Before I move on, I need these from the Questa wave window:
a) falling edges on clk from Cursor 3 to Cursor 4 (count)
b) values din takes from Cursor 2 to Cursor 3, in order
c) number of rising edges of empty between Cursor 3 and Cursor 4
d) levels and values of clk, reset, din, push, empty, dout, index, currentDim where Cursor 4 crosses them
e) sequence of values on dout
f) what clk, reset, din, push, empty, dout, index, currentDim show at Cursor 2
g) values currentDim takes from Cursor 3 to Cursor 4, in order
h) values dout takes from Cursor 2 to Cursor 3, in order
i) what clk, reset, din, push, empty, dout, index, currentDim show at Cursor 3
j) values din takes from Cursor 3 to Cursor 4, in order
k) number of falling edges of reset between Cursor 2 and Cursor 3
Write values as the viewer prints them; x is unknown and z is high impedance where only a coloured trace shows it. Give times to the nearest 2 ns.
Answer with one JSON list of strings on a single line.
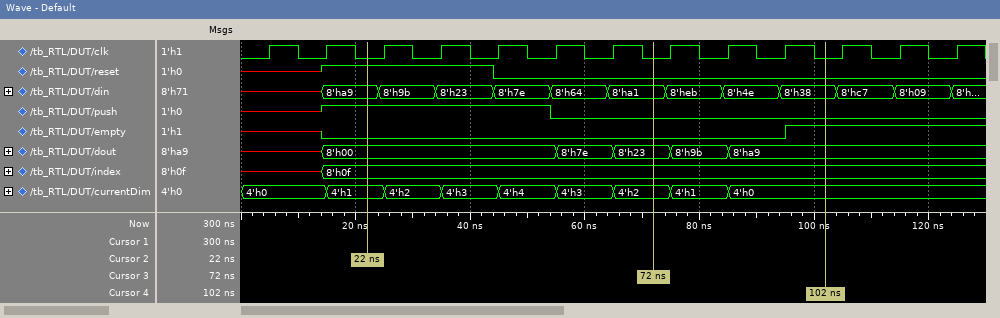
["3", "8'ha9, 8'h9b, 8'h23, 8'h7e, 8'h64, 8'ha1", "1", "clk=0, reset=0, din=8'h38, push=0, empty=1, dout=8'ha9, index=8'h0f, currentDim=4'h0", "x, 8'h00, 8'h7e, 8'h23, 8'h9b, 8'ha9", "clk=0, reset=1, din=8'ha9, push=1, empty=0, dout=8'h00, index=8'h0f, currentDim=4'h1", "4'h2, 4'h1, 4'h0", "8'h00, 8'h7e, 8'h23", "clk=0, reset=0, din=8'ha1, push=0, empty=0, dout=8'h23, index=8'h0f, currentDim=4'h2", "8'ha1, 8'heb, 8'h4e, 8'h38", "1"]
